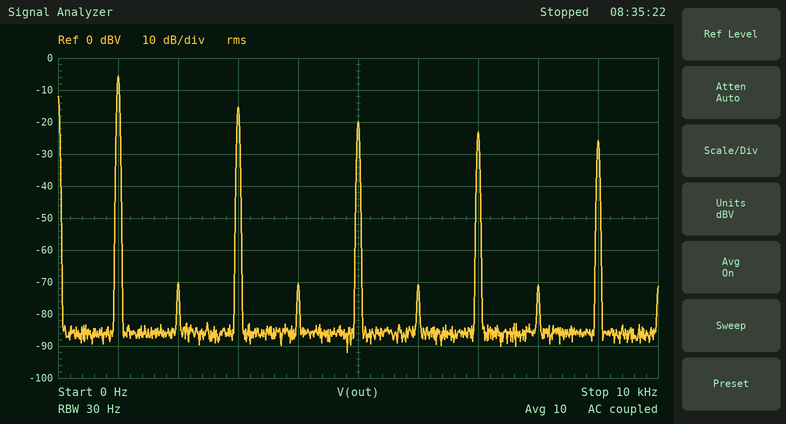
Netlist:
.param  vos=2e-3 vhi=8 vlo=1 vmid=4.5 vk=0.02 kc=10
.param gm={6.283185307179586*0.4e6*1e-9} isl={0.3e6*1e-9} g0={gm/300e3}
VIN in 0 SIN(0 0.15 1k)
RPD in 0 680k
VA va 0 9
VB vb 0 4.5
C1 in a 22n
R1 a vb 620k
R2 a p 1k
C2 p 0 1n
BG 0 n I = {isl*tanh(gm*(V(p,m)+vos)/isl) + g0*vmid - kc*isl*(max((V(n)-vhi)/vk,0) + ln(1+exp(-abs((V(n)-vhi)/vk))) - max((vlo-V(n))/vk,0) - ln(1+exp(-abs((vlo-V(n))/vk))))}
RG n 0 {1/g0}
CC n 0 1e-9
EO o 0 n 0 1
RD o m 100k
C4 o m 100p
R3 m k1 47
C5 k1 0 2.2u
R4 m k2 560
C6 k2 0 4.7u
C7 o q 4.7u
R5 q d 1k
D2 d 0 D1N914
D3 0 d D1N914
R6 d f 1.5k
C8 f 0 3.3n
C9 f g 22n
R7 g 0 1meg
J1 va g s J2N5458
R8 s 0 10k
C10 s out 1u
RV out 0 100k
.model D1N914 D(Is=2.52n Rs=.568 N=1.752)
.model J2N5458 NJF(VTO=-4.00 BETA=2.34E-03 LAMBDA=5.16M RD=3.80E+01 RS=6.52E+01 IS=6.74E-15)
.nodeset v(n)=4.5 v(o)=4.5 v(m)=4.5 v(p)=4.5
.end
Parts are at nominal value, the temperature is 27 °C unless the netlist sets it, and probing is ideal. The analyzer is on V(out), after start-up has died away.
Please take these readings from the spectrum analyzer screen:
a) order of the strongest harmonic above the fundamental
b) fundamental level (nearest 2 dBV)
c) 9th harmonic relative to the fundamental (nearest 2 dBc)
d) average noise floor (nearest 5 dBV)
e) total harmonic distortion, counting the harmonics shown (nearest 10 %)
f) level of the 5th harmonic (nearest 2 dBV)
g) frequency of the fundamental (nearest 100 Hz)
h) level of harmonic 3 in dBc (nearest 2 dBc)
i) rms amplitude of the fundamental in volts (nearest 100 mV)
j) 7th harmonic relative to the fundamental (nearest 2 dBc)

3
-6 dBV
-20 dBc
-85 dBV
40 %
-20 dBV
1.0 kHz
-10 dBc
500 mV
-18 dBc
